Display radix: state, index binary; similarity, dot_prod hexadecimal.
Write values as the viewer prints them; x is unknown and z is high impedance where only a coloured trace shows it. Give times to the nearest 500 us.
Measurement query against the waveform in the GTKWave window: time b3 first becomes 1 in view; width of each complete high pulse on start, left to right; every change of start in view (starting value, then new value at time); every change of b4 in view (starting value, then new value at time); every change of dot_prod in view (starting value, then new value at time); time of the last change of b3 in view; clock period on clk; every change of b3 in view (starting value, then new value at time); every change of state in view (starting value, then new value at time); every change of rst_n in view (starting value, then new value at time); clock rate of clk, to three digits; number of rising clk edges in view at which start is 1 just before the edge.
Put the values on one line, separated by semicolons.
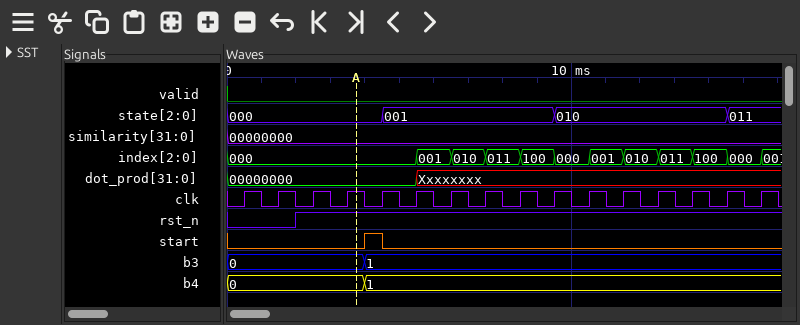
4000 us; 500 us; 0, 1 at 4000 us, 0 at 4500 us; 0, 1 at 4000 us; 00000000, Xxxxxxxx at 5500 us; 4000 us; 1000 us; 0, 1 at 4000 us; 000, 001 at 4500 us, 010 at 9500 us, 011 at 14500 us; 0, 1 at 2000 us; 1.00 kHz; 1
